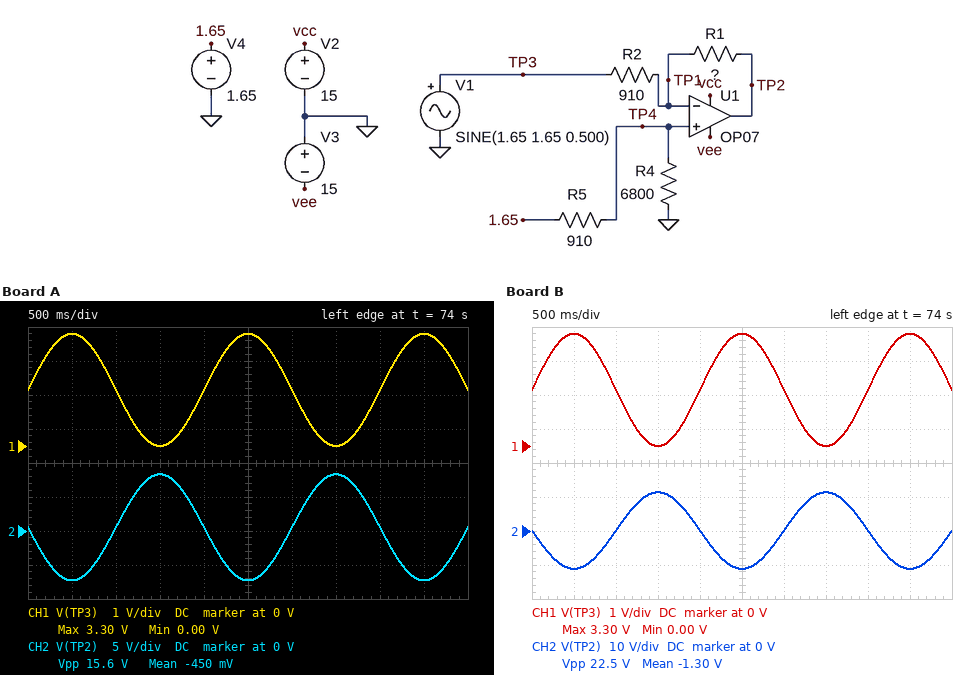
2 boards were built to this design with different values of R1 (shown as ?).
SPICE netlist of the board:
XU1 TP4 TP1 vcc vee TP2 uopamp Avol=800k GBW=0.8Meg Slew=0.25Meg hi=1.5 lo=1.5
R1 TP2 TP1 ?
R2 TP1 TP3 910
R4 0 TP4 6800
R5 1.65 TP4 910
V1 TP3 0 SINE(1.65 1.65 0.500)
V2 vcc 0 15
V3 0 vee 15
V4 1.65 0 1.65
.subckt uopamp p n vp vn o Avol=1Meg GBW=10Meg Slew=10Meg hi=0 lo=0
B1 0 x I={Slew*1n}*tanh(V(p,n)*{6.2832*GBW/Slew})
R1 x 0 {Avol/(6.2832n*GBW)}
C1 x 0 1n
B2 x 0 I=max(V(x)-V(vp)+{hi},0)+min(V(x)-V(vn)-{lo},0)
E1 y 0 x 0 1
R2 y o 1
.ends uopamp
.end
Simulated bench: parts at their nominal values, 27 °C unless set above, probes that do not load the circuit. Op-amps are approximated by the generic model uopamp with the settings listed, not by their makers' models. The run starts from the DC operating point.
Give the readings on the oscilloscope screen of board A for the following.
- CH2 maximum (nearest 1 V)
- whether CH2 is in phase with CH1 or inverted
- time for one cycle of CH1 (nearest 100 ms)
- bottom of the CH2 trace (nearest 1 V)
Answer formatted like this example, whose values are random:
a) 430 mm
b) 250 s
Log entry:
a) 8 V
b) inverted
c) 2.0 s
d) -7 V
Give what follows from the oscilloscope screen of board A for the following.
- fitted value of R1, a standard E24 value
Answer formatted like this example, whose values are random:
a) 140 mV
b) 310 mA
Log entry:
a) 4.3 kΩ
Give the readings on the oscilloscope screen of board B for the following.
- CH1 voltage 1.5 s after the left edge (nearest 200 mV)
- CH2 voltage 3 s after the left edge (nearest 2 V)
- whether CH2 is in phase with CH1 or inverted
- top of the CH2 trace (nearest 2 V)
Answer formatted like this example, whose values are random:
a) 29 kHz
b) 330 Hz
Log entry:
a) 0 V
b) 0 V
c) inverted
d) 12 V
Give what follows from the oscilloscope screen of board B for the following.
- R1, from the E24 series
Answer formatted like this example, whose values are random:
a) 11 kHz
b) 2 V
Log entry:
a) 6.2 kΩ
